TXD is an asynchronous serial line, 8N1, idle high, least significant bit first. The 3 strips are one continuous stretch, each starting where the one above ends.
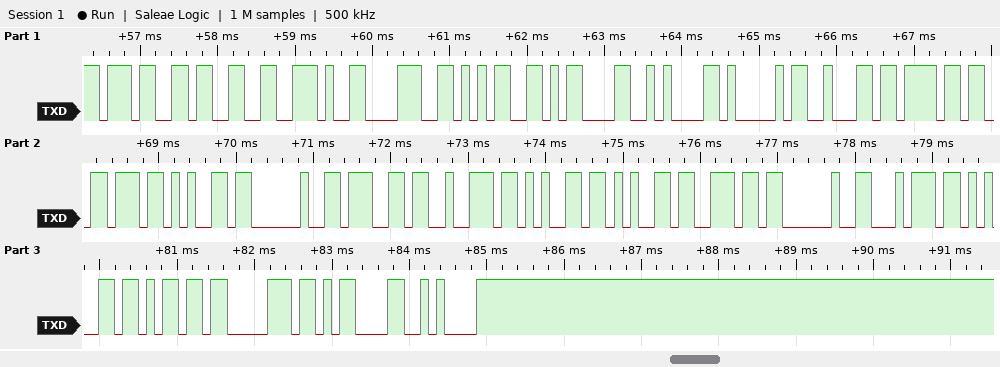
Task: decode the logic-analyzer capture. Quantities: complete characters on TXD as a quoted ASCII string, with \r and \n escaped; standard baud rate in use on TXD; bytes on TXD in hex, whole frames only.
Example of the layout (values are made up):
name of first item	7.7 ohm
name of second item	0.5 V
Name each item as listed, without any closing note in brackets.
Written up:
complete characters on TXD as a quoted ASCII string, with \r and \n escaped	"73.85\r\nAbove green temp\r\n"
standard baud rate in use on TXD	9600 baud
bytes on TXD in hex, whole frames only	37 33 2E 38 35 0D 0A 41 62 6F 76 65 20 67 72 65 65 6E 20 74 65 6D 70 0D 0A
